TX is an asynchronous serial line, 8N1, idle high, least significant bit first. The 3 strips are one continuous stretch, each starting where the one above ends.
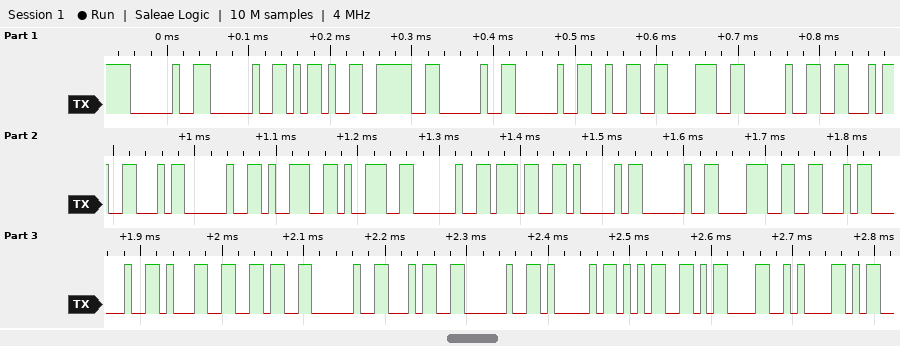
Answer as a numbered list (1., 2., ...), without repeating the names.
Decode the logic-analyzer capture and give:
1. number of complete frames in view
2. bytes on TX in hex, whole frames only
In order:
1. 30
2. 20 20 2D 3E 20 20 32 38 20 46 46 20 39 39 20 37 41 20 38 46 20 31 36 20 34 20 41 35 0D 0A
